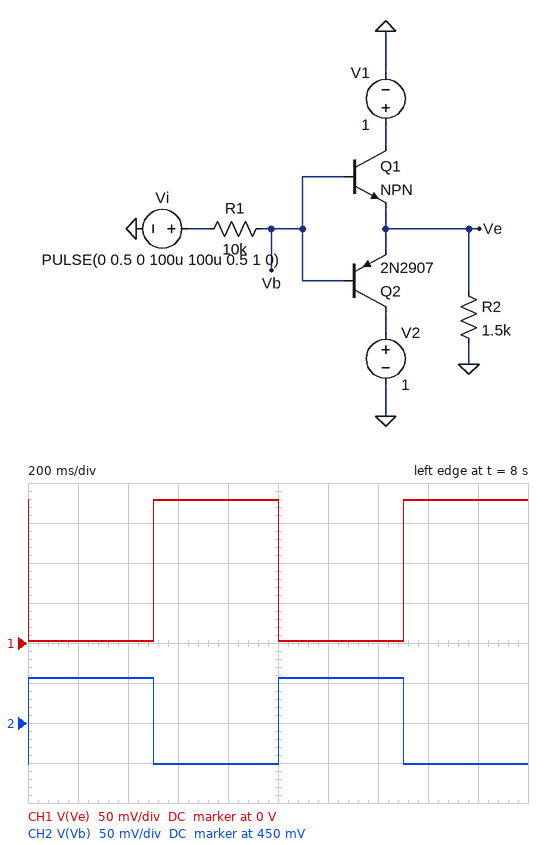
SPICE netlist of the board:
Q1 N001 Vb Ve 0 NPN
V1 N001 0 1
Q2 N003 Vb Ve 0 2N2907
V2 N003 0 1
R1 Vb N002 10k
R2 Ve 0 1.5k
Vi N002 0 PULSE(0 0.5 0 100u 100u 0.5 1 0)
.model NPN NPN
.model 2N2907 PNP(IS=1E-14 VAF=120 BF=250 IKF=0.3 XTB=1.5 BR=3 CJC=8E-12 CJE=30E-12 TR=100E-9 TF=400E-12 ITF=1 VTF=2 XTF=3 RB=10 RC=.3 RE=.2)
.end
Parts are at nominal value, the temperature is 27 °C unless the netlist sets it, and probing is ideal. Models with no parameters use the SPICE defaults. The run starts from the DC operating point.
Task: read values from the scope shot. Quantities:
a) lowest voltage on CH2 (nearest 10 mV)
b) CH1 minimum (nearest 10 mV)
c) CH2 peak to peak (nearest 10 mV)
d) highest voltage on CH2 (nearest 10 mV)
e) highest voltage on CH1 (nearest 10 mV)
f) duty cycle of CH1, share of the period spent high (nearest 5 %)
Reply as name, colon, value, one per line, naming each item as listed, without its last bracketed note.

lowest voltage on CH2: 400 mV
CH1 minimum: 0 V
CH2 peak to peak: 110 mV
highest voltage on CH2: 510 mV
highest voltage on CH1: 180 mV
duty cycle of CH1, share of the period spent high: 50 %
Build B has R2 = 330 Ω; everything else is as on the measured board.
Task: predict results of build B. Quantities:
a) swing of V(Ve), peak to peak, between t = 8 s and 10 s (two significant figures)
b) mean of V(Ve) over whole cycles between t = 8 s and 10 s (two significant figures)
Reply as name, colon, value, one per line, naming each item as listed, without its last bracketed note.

swing of V(Ve), peak to peak, between t = 8 s and 10 s: 39 mV
mean of V(Ve) over whole cycles between t = 8 s and 10 s: 20 mV
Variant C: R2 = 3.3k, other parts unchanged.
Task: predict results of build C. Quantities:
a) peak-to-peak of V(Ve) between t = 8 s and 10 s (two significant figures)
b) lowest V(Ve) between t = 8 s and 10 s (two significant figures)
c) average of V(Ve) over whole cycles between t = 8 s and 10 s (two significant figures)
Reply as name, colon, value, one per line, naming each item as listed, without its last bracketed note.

peak-to-peak of V(Ve) between t = 8 s and 10 s: 390 mV
lowest V(Ve) between t = 8 s and 10 s: 6.4 mV
average of V(Ve) over whole cycles between t = 8 s and 10 s: 200 mV
